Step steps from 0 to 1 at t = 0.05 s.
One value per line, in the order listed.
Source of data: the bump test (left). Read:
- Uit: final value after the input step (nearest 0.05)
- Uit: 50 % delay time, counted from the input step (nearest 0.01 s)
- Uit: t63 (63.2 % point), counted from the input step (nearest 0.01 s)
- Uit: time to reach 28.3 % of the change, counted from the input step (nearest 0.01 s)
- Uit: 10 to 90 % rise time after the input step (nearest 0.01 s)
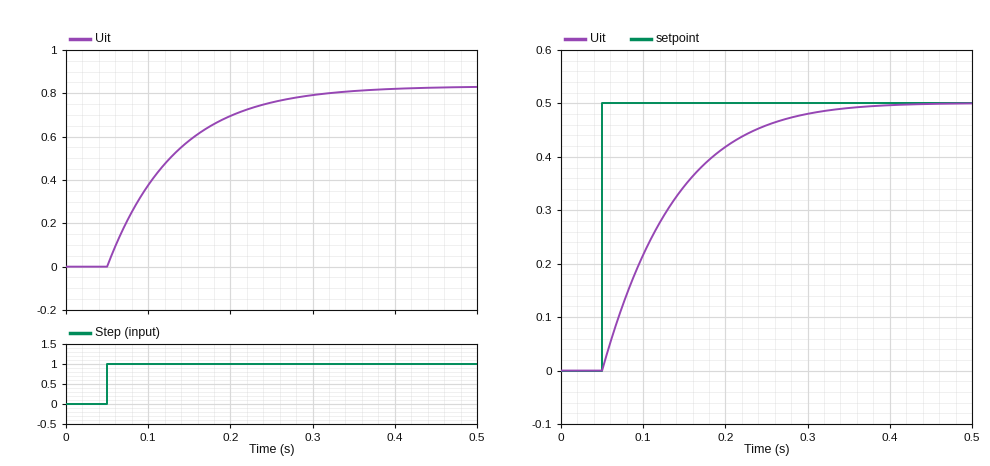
0.85
0.06 s
0.08 s
0.03 s
0.18 s
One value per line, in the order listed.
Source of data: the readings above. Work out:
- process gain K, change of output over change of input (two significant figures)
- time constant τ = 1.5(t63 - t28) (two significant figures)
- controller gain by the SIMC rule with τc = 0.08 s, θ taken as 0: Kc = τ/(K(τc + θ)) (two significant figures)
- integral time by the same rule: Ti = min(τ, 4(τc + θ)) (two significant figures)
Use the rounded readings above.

0.85
0.075 s
1.1
0.075 s
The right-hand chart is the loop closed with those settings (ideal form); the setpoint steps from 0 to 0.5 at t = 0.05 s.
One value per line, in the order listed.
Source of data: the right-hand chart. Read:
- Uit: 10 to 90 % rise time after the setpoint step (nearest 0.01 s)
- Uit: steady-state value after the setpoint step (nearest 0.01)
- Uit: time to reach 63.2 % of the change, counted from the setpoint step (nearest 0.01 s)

0.18 s
0.50
0.09 s
